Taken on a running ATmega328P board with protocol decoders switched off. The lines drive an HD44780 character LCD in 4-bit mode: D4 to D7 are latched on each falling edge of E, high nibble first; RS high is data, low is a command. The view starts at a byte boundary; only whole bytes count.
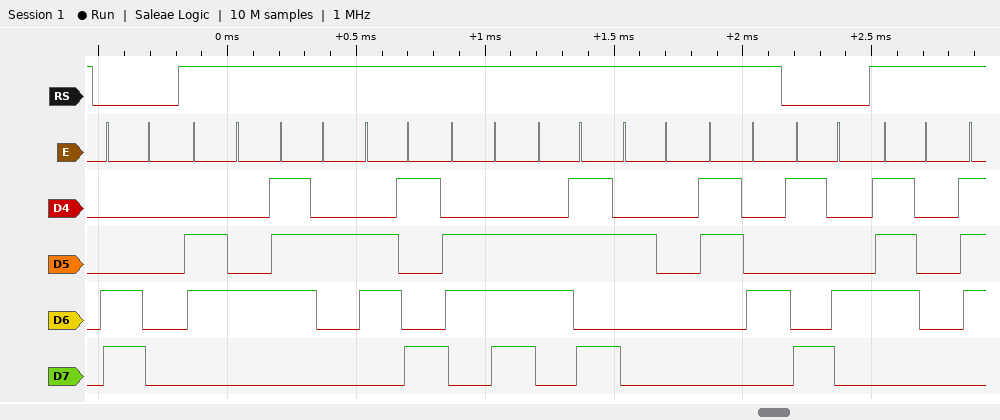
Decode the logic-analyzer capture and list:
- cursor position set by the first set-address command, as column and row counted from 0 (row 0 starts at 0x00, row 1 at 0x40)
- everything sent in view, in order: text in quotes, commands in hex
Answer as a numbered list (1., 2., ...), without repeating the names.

1. column 0, row 1
2. 0xC0 "drink 4" 0x94 "p"
